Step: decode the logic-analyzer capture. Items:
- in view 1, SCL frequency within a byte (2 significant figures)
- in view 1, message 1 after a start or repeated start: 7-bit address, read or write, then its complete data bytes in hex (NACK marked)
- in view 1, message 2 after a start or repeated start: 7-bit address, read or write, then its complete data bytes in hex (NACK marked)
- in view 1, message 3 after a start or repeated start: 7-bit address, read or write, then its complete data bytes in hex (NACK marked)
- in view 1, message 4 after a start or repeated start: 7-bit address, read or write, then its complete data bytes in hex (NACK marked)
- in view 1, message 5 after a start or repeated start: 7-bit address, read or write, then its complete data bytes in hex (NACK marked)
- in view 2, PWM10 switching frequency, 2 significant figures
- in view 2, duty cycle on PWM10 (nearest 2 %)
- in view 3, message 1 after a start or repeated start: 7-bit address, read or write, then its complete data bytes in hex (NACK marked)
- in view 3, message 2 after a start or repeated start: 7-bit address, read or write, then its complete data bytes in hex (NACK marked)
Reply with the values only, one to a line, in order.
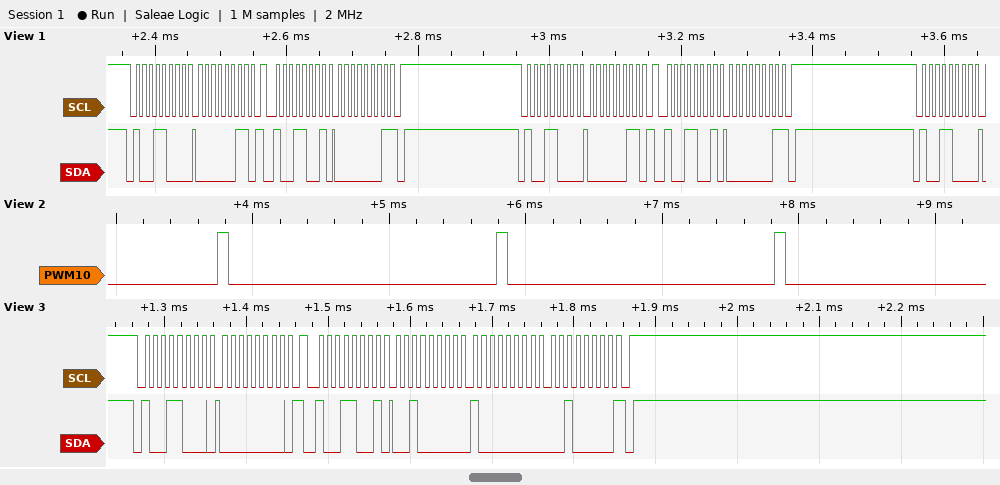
100 kHz
0x4C write: 03
0x4C read: 01 NACK
0x4C write: 03
0x4C read: 01 NACK
0x4C write
490 Hz
4 %
0x4C write: 00
0x4C read: 20 80 20 NACK
